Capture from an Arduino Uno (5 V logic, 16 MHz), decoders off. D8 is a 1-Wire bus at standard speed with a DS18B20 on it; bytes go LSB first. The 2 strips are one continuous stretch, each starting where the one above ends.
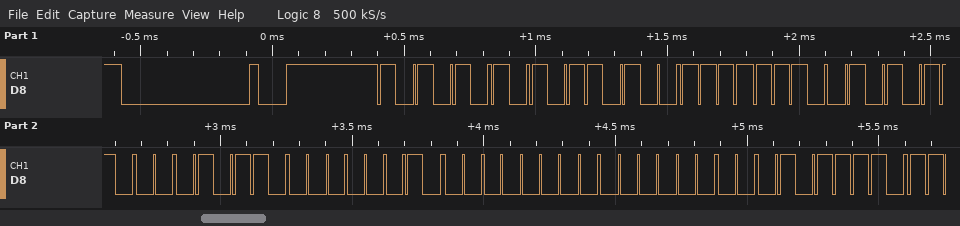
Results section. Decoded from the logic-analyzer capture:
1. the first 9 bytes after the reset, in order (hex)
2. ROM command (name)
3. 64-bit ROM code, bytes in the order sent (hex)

55 2D 7F 6A 68 40 00 00 7A
Match ROM
2D 7F 6A 68 40 00 00 7A
